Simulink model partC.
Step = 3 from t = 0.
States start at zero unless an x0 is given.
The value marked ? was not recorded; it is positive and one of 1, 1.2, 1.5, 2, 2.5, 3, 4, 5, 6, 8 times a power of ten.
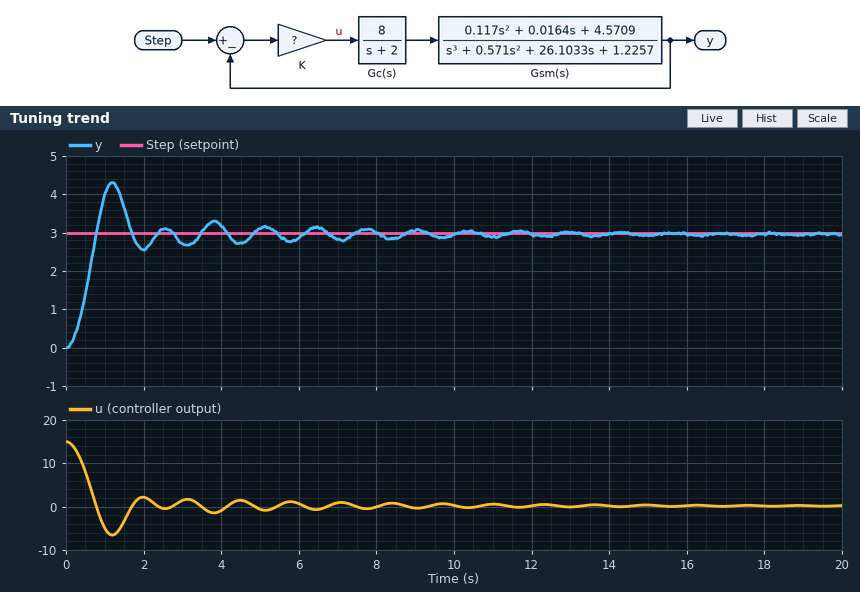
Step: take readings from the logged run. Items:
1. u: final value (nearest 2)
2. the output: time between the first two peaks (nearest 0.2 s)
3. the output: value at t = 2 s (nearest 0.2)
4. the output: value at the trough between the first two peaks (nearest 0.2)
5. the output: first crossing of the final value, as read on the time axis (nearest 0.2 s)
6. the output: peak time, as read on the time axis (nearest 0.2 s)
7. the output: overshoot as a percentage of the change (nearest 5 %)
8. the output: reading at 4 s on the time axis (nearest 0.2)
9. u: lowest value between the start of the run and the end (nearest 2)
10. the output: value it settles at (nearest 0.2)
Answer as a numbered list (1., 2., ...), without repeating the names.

1. 0
2. 1.4 s
3. 2.6
4. 2.6
5. 0.8 s
6. 1.2 s
7. 45 %
8. 3.2
9. -6
10. 3.0
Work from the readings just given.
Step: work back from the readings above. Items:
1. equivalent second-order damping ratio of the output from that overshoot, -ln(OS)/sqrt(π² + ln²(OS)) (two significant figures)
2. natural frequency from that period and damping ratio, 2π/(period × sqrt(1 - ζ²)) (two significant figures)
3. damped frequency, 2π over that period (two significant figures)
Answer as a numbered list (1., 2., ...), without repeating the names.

1. 0.25
2. 4.6 rad/s
3. 4.5 rad/s
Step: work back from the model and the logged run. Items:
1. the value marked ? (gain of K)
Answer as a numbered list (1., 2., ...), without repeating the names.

1. 5
